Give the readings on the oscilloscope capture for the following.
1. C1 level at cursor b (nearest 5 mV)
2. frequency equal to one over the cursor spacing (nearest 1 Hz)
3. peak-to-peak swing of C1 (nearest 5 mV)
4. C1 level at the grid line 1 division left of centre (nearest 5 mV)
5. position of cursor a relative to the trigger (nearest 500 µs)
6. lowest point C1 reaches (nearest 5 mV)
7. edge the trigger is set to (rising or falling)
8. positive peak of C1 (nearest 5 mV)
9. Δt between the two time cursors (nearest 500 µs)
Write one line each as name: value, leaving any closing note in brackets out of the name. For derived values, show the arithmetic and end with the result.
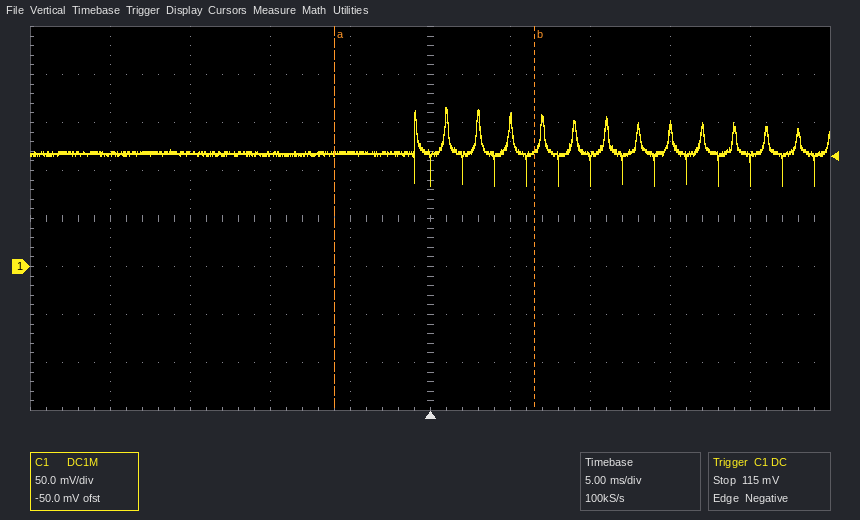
C1 level at cursor b: 120 mV
frequency equal to one over the cursor spacing: 1 / 12.5 ms ≈ 80 Hz
peak-to-peak swing of C1: 165 mV − (85 mV) = 80 mV
C1 level at the grid line 1 division left of centre: 120 mV
position of cursor a relative to the trigger: -6.0 ms
lowest point C1 reaches: 85 mV
edge the trigger is set to: falling
positive peak of C1: 165 mV
Δt between the two time cursors: 12.5 ms
